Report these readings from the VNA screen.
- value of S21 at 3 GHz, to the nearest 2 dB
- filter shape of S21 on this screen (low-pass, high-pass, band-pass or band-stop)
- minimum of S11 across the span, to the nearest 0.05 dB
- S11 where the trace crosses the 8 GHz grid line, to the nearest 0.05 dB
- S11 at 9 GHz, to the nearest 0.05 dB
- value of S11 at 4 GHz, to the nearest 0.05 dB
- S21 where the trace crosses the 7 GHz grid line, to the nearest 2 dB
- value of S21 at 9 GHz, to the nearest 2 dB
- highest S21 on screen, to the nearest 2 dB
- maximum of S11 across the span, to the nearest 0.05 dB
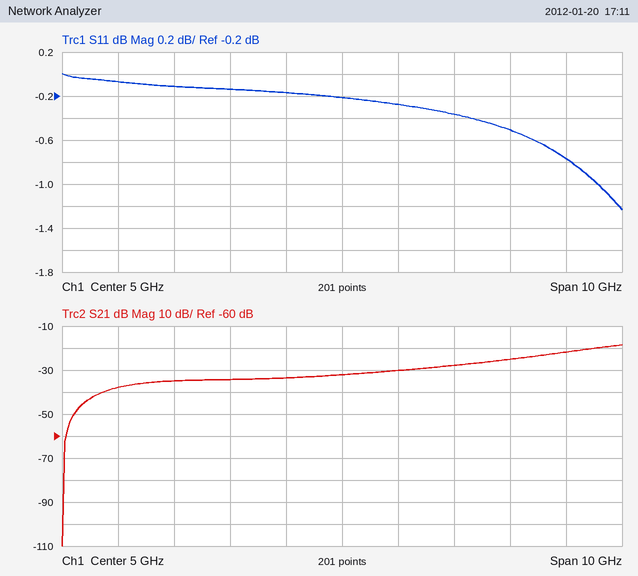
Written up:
-34 dB
high-pass
-1.25 dB
-0.50 dB
-0.75 dB
-0.15 dB
-28 dB
-22 dB
-18 dB
0.00 dB
